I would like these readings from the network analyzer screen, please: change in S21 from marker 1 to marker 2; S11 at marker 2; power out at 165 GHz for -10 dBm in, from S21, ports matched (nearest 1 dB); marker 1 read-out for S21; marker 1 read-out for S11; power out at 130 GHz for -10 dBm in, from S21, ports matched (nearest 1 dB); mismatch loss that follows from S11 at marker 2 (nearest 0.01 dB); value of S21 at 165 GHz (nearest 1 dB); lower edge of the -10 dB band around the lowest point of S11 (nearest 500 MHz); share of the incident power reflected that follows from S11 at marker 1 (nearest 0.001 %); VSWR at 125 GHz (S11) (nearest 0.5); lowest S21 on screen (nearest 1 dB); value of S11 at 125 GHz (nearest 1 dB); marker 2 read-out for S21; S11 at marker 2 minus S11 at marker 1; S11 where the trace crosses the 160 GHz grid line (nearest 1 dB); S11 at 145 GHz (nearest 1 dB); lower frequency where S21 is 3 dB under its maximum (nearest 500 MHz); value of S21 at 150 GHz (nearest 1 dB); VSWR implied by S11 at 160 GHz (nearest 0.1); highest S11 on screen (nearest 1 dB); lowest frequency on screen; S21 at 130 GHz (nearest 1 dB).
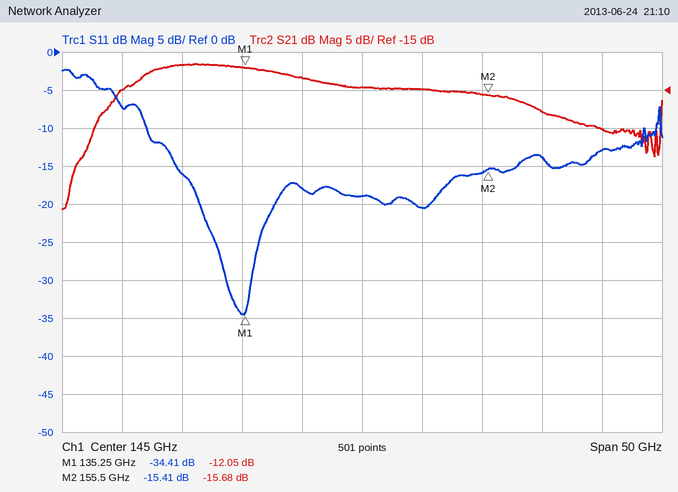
-3.63 dB
-15.41 dB
-30 dBm
-12.05 dB
-34.41 dB
-22 dBm
0.13 dB
-20 dB
127.0 GHz
0.036 %
2.5
-31 dB
-7 dB
-15.68 dB
19.00 dB
-14 dB
-19 dB
125.5 GHz
-15 dB
1.5
-2 dB
120 GHz
-12 dB
